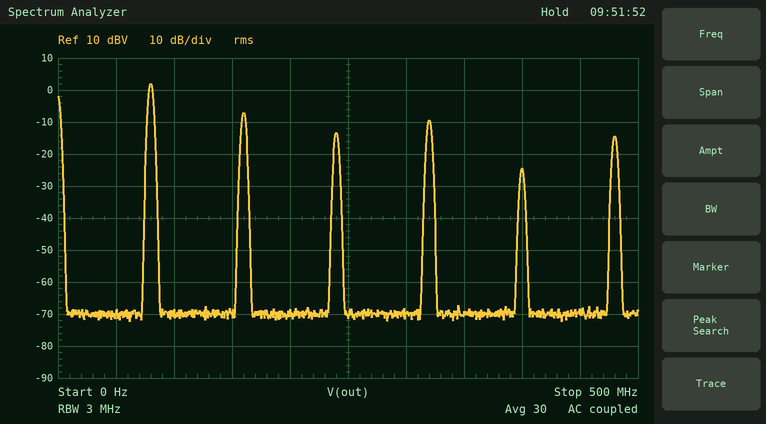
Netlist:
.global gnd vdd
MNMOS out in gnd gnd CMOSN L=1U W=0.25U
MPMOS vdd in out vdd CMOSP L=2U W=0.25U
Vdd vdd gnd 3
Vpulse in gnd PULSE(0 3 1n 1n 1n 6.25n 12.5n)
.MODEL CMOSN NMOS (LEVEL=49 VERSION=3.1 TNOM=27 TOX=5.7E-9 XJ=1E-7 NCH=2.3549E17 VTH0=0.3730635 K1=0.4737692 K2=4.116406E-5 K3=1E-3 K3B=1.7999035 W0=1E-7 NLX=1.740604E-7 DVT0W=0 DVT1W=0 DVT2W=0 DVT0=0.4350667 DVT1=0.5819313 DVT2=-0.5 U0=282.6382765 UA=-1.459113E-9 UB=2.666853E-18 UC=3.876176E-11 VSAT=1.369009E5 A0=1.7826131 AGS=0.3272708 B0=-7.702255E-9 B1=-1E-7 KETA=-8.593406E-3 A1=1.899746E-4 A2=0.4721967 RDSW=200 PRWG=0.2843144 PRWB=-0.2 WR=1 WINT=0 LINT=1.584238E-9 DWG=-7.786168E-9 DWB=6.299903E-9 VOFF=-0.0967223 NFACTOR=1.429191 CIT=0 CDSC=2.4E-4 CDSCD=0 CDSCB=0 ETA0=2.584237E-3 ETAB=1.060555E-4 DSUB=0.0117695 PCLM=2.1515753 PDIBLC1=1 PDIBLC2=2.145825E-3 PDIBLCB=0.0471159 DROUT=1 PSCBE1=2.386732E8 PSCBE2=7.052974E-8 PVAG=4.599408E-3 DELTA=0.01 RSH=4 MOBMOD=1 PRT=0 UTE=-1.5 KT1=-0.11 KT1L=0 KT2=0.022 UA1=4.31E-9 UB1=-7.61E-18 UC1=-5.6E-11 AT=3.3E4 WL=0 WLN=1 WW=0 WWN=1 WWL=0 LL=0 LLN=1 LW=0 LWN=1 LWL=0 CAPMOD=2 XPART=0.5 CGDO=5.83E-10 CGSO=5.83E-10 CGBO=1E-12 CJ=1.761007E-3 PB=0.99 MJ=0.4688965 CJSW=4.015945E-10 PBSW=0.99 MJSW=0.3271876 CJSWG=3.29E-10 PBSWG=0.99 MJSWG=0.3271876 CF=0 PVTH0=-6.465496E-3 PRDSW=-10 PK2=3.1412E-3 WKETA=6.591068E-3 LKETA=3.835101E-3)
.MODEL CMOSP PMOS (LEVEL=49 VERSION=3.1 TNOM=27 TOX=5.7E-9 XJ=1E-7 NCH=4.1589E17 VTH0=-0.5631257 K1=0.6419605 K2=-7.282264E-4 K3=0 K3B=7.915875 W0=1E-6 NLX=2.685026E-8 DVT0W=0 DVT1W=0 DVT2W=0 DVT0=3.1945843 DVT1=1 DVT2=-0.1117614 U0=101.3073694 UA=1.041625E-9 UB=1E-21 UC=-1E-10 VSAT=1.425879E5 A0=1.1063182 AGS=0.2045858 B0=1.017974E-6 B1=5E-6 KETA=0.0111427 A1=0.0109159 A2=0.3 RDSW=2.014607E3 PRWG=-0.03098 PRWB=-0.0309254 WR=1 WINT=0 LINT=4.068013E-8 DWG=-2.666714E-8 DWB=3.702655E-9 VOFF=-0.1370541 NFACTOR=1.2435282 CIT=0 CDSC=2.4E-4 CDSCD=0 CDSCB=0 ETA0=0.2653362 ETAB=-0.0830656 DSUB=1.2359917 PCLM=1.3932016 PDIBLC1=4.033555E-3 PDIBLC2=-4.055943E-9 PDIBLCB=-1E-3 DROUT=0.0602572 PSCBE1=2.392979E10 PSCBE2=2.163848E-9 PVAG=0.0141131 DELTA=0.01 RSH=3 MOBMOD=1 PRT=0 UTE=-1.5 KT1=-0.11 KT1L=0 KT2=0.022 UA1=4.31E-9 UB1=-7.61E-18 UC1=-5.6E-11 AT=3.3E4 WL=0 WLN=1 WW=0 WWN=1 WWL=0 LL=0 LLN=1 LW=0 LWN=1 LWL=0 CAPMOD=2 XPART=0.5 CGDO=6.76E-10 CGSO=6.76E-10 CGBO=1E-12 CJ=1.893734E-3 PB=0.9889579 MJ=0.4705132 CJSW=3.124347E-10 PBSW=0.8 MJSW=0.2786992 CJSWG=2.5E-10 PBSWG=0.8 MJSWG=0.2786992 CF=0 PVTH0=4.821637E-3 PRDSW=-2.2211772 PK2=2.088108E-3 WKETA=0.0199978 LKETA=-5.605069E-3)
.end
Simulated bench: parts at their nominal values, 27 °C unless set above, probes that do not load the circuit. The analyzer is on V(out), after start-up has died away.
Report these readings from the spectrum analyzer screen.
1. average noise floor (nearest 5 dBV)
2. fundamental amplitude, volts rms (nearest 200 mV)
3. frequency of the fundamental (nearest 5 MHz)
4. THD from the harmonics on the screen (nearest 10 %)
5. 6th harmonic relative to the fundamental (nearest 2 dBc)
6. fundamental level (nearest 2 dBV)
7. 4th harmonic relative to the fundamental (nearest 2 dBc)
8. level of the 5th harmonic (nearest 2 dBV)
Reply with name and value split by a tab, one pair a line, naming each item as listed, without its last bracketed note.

average noise floor	-70 dBV
fundamental amplitude, volts rms	1.2 V
frequency of the fundamental	80 MHz
THD from the harmonics on the screen	50 %
6th harmonic relative to the fundamental	-16 dBc
fundamental level	2 dBV
4th harmonic relative to the fundamental	-12 dBc
level of the 5th harmonic	-24 dBV
